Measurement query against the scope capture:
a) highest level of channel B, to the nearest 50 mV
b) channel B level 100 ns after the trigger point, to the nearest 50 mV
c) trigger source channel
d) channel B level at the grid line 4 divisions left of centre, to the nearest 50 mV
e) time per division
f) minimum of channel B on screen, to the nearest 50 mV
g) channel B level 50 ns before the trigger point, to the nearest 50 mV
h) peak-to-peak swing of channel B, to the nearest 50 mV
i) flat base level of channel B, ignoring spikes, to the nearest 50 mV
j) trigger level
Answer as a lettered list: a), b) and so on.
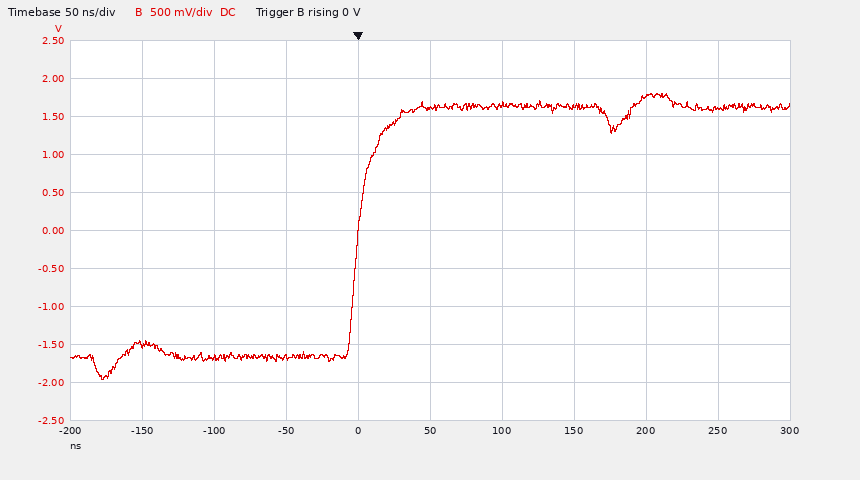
a) 1.80 V
b) 1.65 V
c) channel B
d) -1.50 V
e) 50 ns
f) -1.95 V
g) -1.65 V
h) 3.75 V
i) -1.65 V
j) 0 V
